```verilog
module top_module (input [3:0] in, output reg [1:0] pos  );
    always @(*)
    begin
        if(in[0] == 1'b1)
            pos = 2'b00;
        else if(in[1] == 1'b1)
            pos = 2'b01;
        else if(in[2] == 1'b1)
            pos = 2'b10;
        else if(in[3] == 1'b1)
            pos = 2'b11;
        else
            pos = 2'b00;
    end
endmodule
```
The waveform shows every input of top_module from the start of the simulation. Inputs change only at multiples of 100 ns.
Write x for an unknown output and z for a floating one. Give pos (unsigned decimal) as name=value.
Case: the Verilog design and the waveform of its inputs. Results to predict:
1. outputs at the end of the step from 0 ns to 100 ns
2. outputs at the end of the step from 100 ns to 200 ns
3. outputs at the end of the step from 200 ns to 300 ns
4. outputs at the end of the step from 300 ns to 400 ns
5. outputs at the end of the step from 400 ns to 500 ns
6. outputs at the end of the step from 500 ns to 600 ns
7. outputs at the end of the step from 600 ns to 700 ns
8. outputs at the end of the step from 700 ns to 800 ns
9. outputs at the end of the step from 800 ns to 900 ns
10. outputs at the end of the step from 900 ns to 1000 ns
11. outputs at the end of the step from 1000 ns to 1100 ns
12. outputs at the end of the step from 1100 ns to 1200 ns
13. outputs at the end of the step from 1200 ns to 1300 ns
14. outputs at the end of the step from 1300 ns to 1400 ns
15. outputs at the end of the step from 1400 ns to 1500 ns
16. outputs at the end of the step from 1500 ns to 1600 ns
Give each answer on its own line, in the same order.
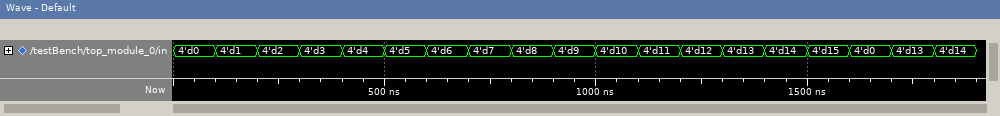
pos=0
pos=0
pos=1
pos=0
pos=2
pos=0
pos=1
pos=0
pos=3
pos=0
pos=1
pos=0
pos=2
pos=0
pos=1
pos=0
